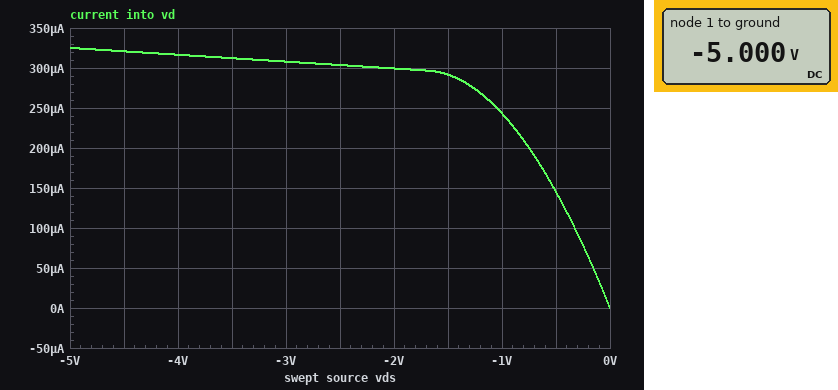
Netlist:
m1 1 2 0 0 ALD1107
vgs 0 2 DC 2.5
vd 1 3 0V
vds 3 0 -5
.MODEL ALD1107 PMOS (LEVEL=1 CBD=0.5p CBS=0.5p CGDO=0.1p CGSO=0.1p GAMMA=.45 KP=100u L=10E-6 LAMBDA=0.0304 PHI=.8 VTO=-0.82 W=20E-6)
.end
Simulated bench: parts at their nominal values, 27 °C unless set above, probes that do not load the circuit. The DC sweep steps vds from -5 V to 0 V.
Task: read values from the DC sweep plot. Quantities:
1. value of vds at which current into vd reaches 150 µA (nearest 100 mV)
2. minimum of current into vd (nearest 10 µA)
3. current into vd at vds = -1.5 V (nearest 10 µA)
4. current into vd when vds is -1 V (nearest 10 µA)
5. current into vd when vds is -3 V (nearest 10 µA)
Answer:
-500 mV
0 A
290 µA
240 µA
310 µA
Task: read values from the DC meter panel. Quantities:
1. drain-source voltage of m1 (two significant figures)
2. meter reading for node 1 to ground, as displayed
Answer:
-5.0 V
-5.000 V
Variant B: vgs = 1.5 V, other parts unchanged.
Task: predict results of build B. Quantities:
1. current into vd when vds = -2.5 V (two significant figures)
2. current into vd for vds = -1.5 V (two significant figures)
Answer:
50 µA
48 µA
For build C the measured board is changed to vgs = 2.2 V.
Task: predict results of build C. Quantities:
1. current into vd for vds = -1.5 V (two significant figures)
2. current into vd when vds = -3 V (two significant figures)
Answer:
200 µA
210 µA
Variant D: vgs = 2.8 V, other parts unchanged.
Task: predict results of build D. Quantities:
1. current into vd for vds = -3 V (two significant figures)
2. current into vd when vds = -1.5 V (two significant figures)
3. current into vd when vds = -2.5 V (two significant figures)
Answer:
430 µA
390 µA
420 µA
